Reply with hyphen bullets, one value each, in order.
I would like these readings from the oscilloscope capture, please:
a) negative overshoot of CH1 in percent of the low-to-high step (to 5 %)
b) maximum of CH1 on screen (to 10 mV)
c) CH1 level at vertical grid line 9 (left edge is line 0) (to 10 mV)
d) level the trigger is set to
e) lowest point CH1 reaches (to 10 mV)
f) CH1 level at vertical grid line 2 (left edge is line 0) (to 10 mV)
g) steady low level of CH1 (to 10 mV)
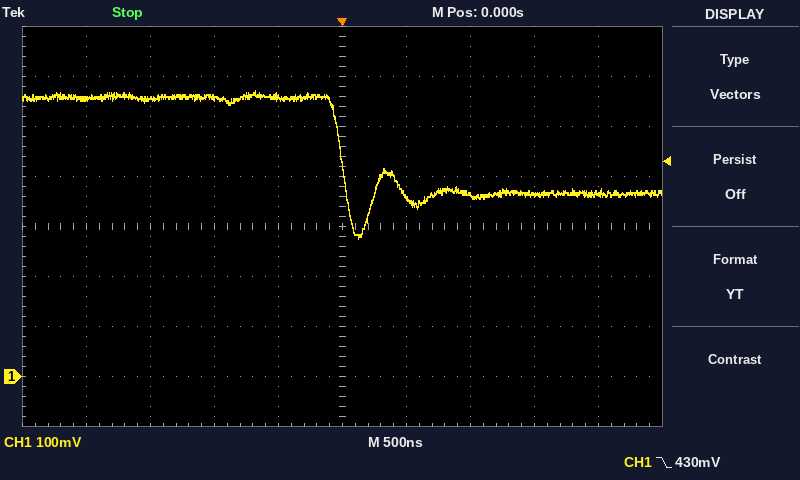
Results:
- 45 %
- 570 mV
- 370 mV
- 430 mV
- 280 mV
- 560 mV
- 370 mV
